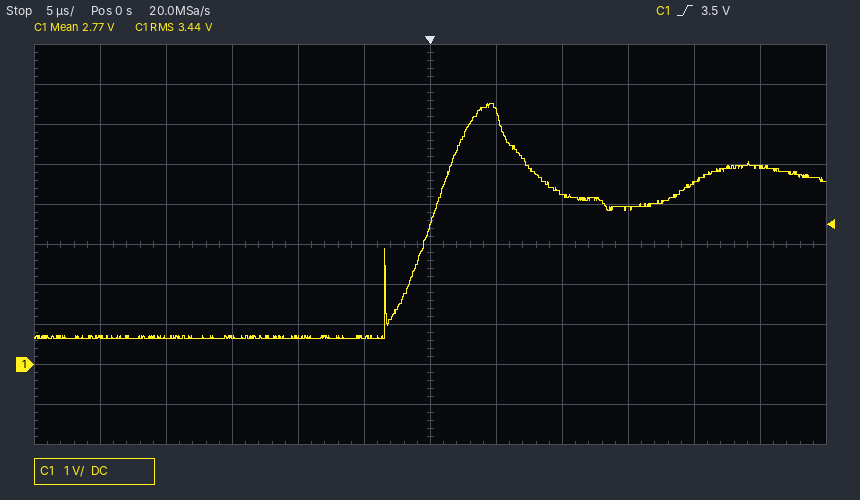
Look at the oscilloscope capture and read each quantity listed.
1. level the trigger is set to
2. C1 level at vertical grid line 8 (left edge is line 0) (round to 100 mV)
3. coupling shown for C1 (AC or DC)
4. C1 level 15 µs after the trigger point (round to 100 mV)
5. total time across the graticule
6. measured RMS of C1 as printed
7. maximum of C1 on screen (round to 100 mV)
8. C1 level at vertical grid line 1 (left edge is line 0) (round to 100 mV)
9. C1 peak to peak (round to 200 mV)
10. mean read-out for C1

3.5 V
4.3 V
DC
3.9 V
60 µs
3.44 V
6.5 V
700 mV
5.8 V
2.77 V
